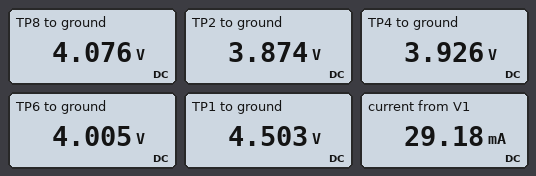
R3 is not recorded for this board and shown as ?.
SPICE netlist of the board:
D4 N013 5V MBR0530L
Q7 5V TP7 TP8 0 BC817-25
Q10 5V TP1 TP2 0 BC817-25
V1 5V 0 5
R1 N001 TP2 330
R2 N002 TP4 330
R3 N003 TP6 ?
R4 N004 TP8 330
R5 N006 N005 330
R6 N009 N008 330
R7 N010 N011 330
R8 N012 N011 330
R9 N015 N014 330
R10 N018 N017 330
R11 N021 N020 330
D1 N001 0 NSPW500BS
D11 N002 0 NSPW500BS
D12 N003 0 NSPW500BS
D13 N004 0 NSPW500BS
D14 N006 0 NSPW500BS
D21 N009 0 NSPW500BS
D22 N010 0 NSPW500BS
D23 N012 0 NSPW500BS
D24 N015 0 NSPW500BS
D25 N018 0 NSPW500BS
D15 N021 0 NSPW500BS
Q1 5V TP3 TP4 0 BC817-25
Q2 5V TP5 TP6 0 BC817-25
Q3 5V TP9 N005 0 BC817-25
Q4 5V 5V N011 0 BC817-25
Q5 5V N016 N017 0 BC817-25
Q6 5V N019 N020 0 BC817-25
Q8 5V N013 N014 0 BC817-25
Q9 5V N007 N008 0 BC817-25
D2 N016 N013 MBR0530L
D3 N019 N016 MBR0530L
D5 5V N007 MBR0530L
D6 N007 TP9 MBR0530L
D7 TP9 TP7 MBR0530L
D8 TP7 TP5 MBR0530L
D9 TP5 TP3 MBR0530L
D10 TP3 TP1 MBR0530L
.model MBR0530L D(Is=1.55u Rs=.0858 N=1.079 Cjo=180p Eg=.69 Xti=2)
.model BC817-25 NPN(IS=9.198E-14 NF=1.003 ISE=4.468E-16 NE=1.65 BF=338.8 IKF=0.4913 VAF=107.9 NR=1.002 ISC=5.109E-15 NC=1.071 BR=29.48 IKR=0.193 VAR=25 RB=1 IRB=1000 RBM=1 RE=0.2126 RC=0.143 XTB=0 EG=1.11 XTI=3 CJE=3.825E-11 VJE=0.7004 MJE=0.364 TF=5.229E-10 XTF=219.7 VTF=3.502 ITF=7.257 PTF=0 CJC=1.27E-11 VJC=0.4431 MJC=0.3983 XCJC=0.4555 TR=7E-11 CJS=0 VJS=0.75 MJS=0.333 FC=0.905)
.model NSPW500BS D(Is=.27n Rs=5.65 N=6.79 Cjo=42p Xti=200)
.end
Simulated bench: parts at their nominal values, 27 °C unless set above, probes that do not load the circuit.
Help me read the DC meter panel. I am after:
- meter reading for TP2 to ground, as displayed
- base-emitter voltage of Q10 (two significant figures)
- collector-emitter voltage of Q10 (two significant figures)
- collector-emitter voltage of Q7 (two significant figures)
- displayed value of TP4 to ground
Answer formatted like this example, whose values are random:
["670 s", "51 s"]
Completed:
["3.874 V", "630 mV", "1.1 V", "920 mV", "3.926 V"]
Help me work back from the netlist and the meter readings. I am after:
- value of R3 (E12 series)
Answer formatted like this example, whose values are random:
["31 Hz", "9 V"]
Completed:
["470 Ω"]
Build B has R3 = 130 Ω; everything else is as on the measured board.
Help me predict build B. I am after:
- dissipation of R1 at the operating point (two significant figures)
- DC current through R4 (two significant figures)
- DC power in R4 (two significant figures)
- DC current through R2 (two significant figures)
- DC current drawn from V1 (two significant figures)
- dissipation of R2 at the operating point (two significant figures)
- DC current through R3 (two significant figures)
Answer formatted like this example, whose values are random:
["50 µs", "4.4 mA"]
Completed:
["2.9 mW", "3.5 mA", "4.1 mW", "3.1 mA", "33 mA", "3.2 mW", "7.0 mA"]
